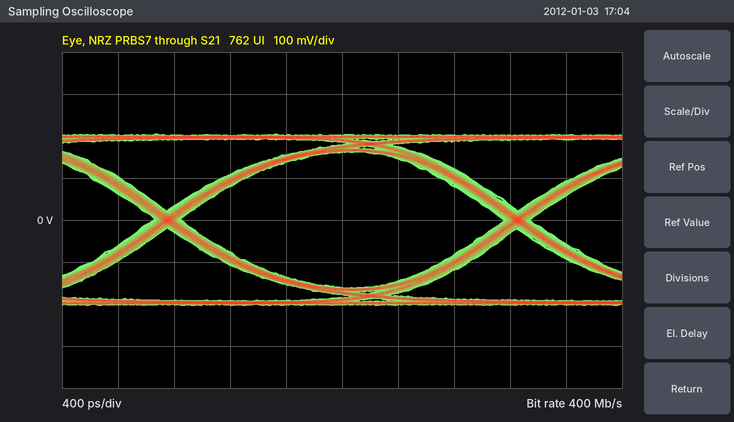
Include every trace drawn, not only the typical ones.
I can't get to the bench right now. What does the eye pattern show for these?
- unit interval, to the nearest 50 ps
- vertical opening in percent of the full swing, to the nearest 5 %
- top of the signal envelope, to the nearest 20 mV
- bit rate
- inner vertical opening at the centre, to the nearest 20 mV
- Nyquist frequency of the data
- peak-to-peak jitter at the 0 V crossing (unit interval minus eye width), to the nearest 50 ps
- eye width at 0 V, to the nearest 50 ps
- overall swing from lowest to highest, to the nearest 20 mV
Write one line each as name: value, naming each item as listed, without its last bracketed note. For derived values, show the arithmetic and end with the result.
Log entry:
unit interval, to the nearest 50 ps: 2.50 ns
vertical opening in percent of the full swing, to the nearest 5 %: 320 mV / 400 mV ≈ 80 %
top of the signal envelope, to the nearest 20 mV: 200 mV
bit rate: 400 Mb/s
inner vertical opening at the centre, to the nearest 20 mV: 320 mV
Nyquist frequency of the data: 200 MHz
peak-to-peak jitter at the 0 V crossing (unit interval minus eye width), to the nearest 50 ps: 200 ps
eye width at 0 V, to the nearest 50 ps: 2.30 ns
overall swing from lowest to highest, to the nearest 20 mV: 400 mV
